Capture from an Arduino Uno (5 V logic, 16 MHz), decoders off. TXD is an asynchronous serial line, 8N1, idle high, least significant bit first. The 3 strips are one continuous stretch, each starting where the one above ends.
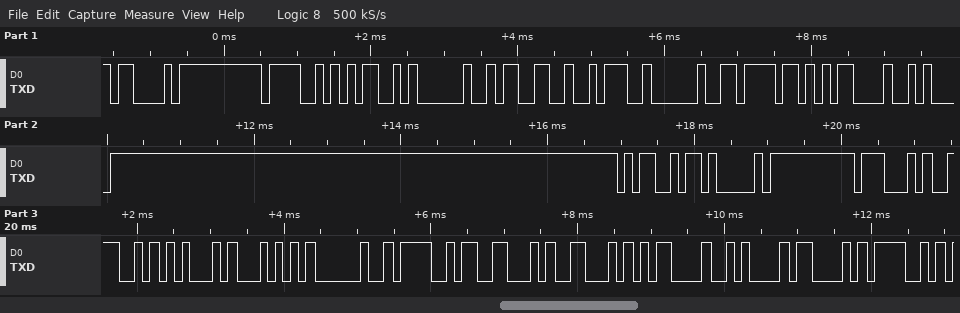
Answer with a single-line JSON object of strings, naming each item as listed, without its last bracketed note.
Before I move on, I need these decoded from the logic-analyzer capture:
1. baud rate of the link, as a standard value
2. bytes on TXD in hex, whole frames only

{"baud rate of the link, as a standard value": "9600 baud", "bytes on TXD in hex, whole frames only": "0x43 0x4F 0x4D 0x20 0x33 0x3A 0x20 0x6F 0x0D 0x0A 0x4D 0x41 0x47 0x4E 0x45 0x54 0x20 0x4F 0x46 0x46 0x0D 0x0A 0x43 0x4F"}
